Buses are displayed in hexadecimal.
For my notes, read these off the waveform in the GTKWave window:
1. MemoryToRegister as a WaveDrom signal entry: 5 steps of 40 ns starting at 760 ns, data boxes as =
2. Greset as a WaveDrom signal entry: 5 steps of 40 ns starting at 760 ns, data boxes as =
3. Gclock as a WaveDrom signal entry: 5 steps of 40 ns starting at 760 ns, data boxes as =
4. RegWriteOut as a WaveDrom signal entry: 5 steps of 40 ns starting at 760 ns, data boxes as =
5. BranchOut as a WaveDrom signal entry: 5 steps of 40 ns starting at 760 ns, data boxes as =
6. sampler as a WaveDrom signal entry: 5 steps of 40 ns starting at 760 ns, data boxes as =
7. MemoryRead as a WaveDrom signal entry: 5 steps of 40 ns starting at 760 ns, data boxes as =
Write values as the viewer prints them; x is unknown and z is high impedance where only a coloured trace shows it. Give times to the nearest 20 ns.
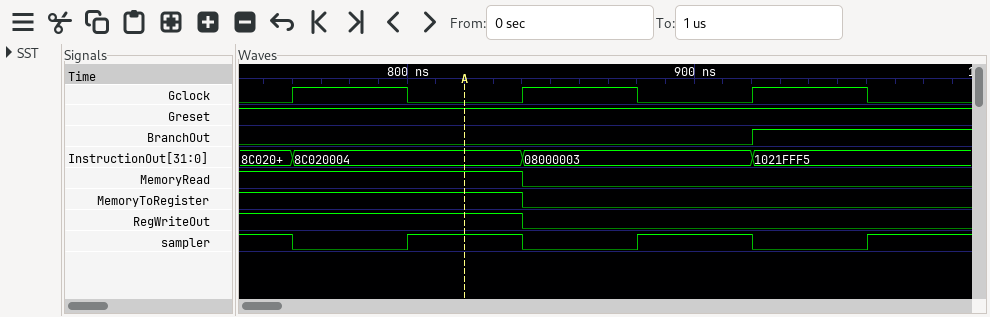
{name: 'MemoryToRegister', wave: '1.0..'}
{name: 'Greset', wave: '1....'}
{name: 'Gclock', wave: '10101'}
{name: 'RegWriteOut', wave: '1.0..'}
{name: 'BranchOut', wave: '0...1'}
{name: 'sampler', wave: '01010'}
{name: 'MemoryRead', wave: '1.0..'}
